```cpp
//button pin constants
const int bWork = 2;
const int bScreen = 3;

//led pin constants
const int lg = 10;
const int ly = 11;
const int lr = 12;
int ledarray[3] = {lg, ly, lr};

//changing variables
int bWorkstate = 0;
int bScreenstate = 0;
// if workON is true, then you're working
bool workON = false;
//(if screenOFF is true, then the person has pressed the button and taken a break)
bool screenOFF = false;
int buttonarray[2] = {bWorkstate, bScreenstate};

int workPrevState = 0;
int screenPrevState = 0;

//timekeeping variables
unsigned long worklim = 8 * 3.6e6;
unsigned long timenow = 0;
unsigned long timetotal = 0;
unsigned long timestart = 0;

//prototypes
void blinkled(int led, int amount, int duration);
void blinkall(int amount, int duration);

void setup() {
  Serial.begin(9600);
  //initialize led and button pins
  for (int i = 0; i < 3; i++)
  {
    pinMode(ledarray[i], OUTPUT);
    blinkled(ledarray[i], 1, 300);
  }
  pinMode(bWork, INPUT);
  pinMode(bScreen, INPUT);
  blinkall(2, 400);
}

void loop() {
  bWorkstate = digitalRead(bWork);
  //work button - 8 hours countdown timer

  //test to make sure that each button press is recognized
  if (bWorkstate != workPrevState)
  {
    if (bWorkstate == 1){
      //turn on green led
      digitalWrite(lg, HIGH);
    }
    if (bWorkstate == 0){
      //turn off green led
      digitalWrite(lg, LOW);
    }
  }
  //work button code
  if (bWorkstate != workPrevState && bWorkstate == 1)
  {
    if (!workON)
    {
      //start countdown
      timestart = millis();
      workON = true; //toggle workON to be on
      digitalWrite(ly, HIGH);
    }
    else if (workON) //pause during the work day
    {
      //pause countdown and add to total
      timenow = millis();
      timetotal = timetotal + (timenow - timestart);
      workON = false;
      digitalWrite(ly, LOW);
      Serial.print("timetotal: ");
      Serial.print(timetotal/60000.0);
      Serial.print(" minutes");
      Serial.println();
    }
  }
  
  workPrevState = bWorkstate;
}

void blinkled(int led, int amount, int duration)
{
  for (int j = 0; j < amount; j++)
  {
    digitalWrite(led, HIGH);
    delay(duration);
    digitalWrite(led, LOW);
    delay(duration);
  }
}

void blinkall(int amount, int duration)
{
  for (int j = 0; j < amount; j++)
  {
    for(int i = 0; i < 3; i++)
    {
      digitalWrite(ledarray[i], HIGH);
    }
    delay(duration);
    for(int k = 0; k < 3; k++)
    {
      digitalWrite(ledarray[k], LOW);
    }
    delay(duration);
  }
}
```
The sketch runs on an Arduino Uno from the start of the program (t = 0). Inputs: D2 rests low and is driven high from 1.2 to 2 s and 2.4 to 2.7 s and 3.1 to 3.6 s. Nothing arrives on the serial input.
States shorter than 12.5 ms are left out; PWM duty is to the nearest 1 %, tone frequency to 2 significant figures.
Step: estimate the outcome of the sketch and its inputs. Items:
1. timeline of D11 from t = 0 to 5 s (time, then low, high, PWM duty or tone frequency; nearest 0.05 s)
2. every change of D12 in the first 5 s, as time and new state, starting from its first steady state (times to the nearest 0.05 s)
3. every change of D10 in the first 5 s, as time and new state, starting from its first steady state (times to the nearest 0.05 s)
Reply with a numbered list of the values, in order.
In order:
1. 0.6 s high; 0.9 s low; 1.8 s high; 2.2 s low; 2.6 s high; 3 s low; 3.4 s high
2. 1.2 s high; 1.5 s low; 1.8 s high; 2.2 s low; 2.6 s high; 3 s low
3. 0 s high; 0.3 s low; 1.8 s high; 2.2 s low; 2.6 s high; 3 s low; 3.4 s high; 3.6 s low
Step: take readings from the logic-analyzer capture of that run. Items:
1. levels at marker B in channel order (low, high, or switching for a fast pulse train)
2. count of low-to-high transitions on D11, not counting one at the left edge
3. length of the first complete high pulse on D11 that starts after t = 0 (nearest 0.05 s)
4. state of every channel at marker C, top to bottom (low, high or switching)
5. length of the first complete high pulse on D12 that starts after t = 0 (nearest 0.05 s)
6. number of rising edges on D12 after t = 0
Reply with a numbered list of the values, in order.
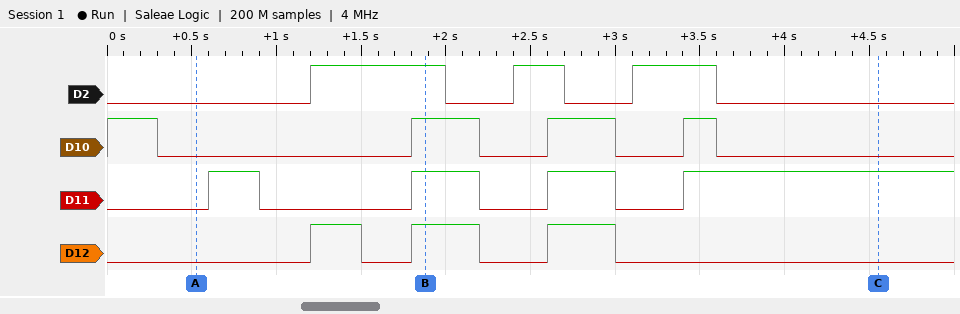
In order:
1. D2 high, D10 high, D11 high, D12 high
2. 4
3. 0.30 s
4. D2 low, D10 low, D11 high, D12 low
5. 0.30 s
6. 3
